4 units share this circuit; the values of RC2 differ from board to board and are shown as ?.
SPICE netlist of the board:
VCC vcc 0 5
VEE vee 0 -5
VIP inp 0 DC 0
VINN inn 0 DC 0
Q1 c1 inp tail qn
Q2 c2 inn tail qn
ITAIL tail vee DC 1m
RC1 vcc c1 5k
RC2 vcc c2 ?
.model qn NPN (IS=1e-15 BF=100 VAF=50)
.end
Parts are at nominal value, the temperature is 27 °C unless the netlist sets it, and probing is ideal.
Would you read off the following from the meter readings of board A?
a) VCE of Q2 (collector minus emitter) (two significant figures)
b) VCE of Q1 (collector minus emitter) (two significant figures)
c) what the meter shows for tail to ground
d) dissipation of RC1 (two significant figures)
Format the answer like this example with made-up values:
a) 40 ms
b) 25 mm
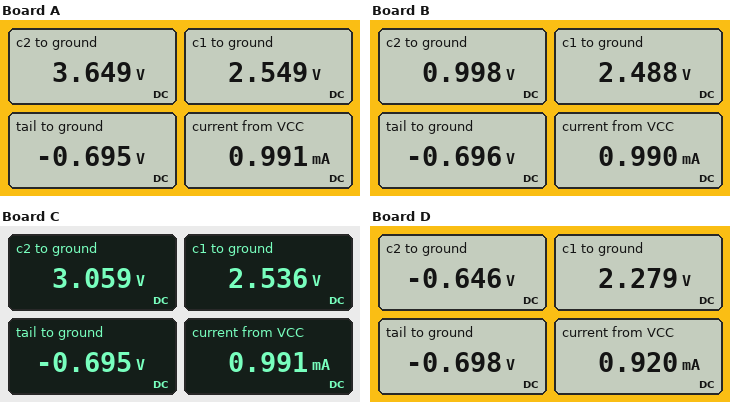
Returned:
a) 4.3 V
b) 3.2 V
c) -0.695 V
d) 1.2 mW
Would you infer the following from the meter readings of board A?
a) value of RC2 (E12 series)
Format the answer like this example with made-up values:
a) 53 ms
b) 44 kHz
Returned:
a) 2.7 kΩ
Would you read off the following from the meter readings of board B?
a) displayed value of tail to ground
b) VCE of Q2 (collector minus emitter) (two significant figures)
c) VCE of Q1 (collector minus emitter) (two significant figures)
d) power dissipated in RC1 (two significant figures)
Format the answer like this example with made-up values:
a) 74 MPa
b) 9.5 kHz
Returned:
a) -0.696 V
b) 1.7 V
c) 3.2 V
d) 1.3 mW
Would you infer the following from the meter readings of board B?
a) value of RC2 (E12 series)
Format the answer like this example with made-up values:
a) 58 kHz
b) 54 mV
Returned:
a) 8.2 kΩ
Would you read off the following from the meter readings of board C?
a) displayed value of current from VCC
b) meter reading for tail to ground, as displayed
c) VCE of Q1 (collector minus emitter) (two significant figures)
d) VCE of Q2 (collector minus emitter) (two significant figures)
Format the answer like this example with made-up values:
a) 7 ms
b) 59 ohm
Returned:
a) 0.991 mA
b) -0.695 V
c) 3.2 V
d) 3.8 V
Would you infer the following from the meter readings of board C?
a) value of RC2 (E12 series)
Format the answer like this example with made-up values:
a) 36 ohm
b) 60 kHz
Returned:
a) 3.9 kΩ
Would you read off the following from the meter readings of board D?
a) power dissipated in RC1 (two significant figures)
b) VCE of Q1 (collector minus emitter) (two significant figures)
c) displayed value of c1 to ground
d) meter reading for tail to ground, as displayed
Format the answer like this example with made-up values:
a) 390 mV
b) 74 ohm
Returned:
a) 1.5 mW
b) 3.0 V
c) 2.279 V
d) -0.698 V
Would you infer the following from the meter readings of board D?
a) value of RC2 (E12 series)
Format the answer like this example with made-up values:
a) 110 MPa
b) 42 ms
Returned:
a) 15 kΩ
